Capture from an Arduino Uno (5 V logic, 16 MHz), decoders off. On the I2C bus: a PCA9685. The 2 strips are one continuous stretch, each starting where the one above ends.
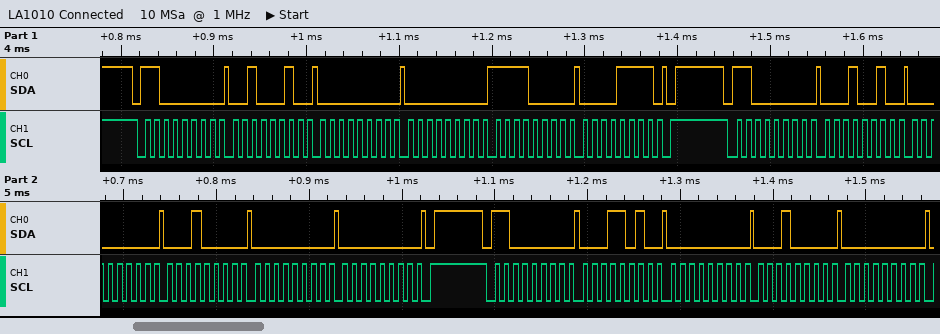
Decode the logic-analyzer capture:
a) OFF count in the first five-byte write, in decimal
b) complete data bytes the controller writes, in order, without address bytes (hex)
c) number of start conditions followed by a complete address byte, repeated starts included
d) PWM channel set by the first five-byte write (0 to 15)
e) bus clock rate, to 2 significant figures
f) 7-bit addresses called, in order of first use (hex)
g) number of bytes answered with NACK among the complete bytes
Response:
4080
22 00 00 F0 0F 12 00 10 00 00 1A 00 10 00
3
7
100 kHz
0x60
0
